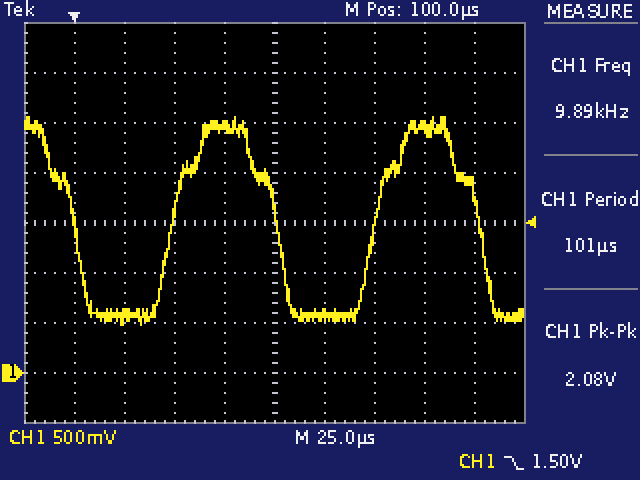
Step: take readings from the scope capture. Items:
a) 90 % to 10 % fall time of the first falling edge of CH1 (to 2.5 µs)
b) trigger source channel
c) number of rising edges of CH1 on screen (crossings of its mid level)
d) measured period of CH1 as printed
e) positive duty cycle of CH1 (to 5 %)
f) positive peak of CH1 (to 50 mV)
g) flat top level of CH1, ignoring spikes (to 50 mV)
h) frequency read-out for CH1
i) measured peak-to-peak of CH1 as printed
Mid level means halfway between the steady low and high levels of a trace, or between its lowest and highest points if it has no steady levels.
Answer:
20.0 µs
CH1
2
101 µs
50 %
2.55 V
2.45 V
9.89 kHz
2.08 V
